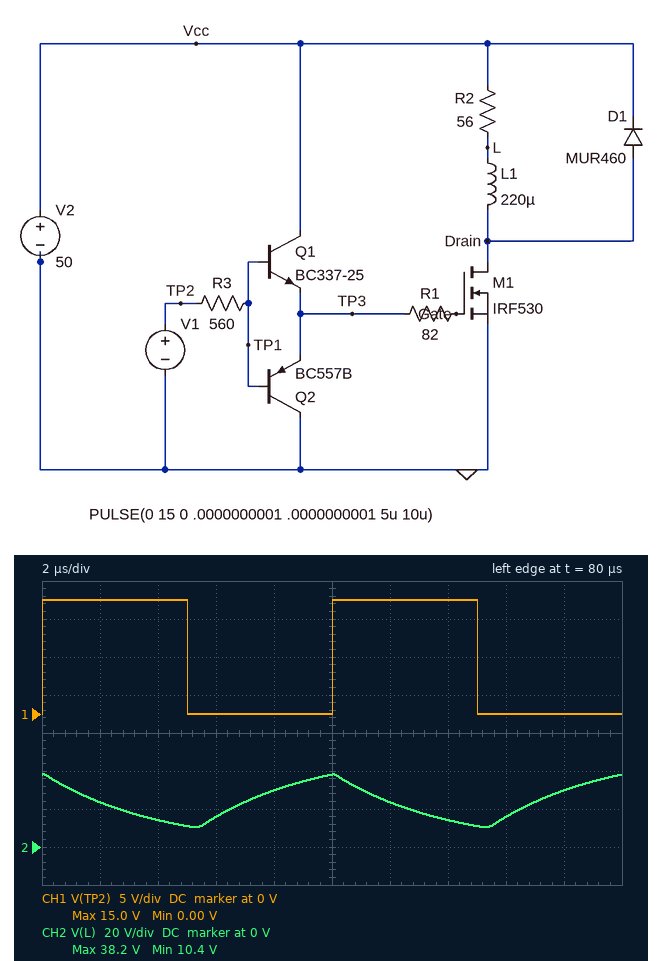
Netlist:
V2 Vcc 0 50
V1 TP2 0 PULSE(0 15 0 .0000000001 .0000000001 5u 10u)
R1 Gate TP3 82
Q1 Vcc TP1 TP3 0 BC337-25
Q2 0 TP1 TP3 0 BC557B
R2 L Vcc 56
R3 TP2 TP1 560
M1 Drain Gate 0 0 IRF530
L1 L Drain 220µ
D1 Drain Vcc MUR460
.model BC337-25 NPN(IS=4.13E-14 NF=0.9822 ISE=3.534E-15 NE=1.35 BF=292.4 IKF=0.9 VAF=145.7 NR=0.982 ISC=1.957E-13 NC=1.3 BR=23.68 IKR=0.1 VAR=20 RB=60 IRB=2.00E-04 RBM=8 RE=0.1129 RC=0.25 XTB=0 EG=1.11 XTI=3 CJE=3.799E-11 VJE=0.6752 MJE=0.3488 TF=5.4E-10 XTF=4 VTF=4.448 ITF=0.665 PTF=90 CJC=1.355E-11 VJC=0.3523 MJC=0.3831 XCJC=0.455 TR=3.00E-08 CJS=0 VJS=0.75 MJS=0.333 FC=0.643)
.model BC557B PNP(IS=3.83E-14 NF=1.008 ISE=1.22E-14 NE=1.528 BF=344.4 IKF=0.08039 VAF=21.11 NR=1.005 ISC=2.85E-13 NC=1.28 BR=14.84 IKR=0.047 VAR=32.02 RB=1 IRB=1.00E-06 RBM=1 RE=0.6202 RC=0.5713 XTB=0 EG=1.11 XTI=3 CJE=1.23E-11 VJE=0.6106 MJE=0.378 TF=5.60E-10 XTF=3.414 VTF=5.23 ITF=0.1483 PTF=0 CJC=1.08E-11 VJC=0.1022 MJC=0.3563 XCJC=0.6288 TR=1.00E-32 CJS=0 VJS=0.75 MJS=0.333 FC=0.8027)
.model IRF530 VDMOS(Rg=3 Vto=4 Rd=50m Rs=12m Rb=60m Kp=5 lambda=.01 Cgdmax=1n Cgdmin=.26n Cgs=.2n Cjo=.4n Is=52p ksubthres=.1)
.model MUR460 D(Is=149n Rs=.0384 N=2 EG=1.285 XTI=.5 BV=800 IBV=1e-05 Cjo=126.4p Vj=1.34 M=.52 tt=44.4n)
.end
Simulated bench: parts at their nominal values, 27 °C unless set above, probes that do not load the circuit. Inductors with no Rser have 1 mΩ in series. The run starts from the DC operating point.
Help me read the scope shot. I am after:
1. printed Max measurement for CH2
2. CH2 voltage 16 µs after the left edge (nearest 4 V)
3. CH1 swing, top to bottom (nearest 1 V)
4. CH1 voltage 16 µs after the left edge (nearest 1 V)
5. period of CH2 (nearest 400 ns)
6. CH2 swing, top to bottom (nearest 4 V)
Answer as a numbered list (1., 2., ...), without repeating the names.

1. 38.2 V
2. 16 V
3. 15 V
4. 0 V
5. 10.0 µs
6. 28 V
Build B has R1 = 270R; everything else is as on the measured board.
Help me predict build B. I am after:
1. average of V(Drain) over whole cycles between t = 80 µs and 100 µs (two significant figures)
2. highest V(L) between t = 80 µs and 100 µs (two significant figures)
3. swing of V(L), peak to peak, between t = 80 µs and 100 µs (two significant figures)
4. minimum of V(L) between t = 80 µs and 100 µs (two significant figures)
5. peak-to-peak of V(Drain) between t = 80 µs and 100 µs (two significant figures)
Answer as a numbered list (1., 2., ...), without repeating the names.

1. 21 V
2. 35 V
3. 26 V
4. 8.9 V
5. 51 V
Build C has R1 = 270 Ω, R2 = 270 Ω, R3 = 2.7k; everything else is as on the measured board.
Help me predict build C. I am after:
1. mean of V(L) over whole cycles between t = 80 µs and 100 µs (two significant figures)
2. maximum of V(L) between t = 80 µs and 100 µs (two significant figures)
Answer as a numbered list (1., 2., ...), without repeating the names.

1. 20 V
2. 50 V
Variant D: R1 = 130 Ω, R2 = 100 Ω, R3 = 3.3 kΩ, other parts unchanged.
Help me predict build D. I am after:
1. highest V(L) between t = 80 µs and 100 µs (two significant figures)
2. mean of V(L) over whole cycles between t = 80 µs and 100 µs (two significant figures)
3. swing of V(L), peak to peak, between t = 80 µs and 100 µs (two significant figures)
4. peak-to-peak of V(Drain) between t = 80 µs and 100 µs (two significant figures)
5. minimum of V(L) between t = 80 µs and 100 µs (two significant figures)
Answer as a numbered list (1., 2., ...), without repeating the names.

1. 44 V
2. 23 V
3. 40 V
4. 51 V
5. 4.3 V
